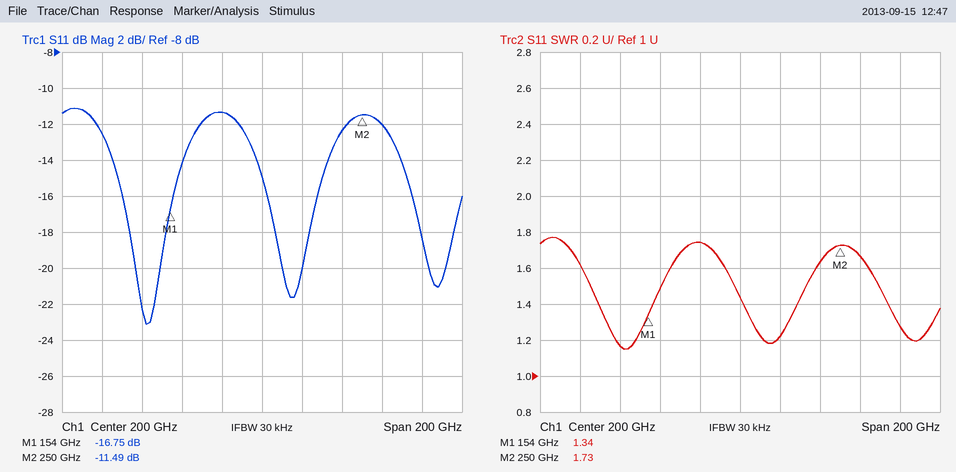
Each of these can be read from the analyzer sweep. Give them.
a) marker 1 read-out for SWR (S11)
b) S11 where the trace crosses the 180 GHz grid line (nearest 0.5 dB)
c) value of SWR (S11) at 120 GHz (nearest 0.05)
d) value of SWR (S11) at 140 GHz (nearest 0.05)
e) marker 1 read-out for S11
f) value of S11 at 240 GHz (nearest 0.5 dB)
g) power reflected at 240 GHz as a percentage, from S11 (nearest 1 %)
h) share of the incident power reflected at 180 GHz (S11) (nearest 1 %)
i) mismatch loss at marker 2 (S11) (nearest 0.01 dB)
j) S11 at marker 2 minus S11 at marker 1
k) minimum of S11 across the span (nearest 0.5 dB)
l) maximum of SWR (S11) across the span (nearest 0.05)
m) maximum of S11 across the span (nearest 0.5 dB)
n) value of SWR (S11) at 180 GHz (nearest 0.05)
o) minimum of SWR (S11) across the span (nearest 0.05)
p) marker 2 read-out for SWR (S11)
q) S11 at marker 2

1.34
-11.5 dB
1.60
1.15
-16.75 dB
-12.5 dB
6 %
7 %
0.32 dB
5.26 dB
-23.0 dB
1.75
-11.0 dB
1.75
1.15
1.73
-11.49 dB
